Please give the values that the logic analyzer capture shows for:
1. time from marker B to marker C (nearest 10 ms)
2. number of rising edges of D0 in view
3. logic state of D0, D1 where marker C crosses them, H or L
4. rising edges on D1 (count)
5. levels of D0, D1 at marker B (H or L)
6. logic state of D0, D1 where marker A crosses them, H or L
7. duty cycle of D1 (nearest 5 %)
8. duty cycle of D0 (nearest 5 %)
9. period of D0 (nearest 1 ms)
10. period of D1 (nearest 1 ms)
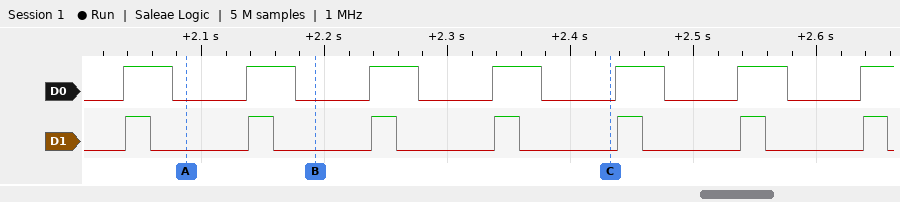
240 ms
7
D0=L, D1=L
7
D0=L, D1=L
D0=L, D1=L
20 %
40 %
100 ms
100 ms
